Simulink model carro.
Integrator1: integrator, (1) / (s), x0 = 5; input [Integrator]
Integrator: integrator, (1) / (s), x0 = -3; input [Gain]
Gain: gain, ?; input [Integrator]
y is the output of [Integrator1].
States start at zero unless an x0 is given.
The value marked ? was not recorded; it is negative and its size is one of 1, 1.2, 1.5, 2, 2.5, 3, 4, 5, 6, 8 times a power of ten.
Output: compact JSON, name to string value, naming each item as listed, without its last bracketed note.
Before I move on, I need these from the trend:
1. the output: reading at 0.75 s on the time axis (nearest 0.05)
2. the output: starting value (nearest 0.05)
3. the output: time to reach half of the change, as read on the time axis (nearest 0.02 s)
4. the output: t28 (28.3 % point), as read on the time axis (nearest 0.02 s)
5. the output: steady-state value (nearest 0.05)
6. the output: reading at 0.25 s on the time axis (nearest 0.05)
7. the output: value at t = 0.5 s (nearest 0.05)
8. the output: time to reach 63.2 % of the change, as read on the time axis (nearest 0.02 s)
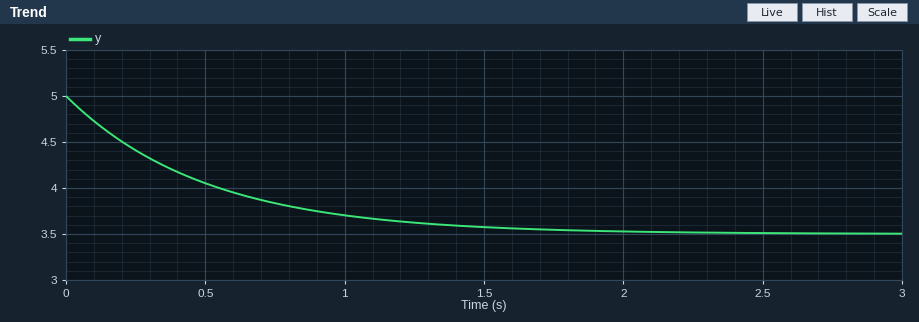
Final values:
{"the output: reading at 0.75 s on the time axis": "3.85", "the output: starting value": "5.00", "the output: time to reach half of the change, as read on the time axis": "0.34 s", "the output: t28 (28.3 % point), as read on the time axis": "0.16 s", "the output: steady-state value": "3.50", "the output: reading at 0.25 s on the time axis": "4.40", "the output: value at t = 0.5 s": "4.05", "the output: time to reach 63.2 % of the change, as read on the time axis": "0.50 s"}
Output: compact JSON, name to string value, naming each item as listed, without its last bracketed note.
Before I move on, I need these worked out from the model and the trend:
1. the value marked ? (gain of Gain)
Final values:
{"the value marked ?": "-2"}
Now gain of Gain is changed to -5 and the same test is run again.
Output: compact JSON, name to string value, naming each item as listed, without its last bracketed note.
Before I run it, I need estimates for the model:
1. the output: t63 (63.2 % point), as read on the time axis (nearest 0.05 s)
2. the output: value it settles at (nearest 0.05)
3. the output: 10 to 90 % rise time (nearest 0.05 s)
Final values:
{"the output: t63 (63.2 % point), as read on the time axis": "0.20 s", "the output: value it settles at": "4.40", "the output: 10 to 90 % rise time": "0.45 s"}
